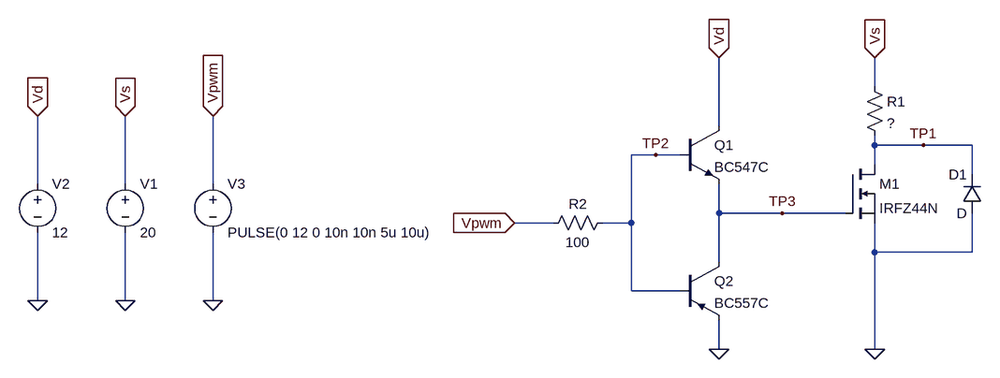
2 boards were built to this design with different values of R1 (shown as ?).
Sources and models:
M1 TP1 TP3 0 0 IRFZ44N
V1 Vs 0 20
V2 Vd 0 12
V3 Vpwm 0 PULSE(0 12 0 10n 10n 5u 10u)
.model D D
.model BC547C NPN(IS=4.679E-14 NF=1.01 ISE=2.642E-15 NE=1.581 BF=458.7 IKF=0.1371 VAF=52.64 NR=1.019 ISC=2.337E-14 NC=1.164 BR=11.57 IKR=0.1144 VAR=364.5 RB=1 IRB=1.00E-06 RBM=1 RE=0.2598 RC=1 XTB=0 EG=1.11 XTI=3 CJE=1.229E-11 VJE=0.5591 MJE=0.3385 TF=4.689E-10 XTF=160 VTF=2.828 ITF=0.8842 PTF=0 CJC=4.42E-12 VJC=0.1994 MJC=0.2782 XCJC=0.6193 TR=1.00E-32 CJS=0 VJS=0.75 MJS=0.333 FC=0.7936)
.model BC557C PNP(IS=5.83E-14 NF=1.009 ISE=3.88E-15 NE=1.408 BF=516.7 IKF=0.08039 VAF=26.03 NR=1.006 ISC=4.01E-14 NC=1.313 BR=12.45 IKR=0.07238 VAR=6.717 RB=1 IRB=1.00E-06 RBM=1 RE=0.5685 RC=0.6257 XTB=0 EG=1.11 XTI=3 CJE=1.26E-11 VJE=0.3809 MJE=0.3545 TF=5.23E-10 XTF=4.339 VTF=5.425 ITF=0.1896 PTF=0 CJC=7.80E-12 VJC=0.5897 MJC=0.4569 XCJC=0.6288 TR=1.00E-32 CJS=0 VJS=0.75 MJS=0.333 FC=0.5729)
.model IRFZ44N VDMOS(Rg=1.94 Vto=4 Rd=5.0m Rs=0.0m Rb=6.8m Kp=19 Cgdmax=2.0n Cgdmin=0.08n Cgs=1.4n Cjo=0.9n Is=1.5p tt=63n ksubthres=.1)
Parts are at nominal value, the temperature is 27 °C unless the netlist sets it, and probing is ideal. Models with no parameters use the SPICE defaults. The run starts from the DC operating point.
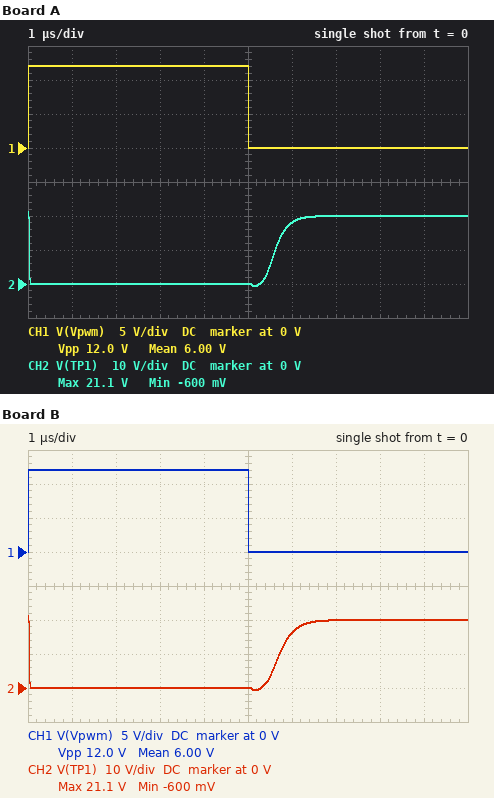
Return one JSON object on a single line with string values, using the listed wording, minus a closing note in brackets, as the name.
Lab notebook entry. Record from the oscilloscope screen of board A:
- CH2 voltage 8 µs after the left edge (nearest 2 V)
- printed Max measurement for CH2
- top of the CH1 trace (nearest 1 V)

{"CH2 voltage 8 µs after the left edge": "20 V", "printed Max measurement for CH2": "21.1 V", "top of the CH1 trace": "12 V"}
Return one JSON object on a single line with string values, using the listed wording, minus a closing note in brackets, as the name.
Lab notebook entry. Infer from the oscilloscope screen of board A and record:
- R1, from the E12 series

{"R1, from the E12 series": "680 Ω"}
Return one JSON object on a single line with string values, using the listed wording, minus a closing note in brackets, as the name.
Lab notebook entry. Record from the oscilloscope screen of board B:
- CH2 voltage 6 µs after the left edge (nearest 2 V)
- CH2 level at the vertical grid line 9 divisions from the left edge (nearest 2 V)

{"CH2 voltage 6 µs after the left edge": "16 V", "CH2 level at the vertical grid line 9 divisions from the left edge": "20 V"}
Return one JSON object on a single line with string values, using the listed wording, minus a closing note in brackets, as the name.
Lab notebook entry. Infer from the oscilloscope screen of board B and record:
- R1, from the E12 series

{"R1, from the E12 series": "820 Ω"}
